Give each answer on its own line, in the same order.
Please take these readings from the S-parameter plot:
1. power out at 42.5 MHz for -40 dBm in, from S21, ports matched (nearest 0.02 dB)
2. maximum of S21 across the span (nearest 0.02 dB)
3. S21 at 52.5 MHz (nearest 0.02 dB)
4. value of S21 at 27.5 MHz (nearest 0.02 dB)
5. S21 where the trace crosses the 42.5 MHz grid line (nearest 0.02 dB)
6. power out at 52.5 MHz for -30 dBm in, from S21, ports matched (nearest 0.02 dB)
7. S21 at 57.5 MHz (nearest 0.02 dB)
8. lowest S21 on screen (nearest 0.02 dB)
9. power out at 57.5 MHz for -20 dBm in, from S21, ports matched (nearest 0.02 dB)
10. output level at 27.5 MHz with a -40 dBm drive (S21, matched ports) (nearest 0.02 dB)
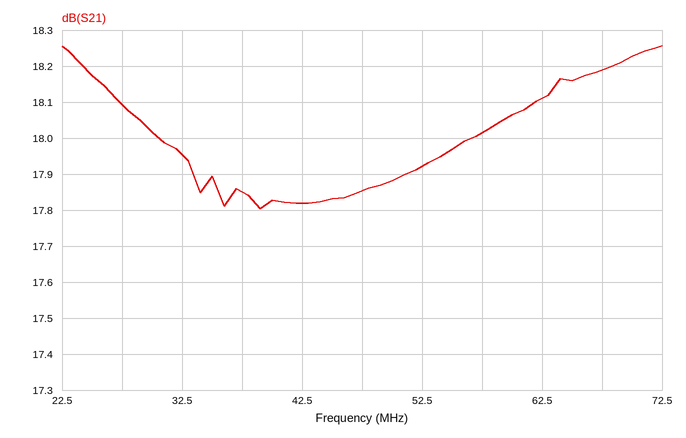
-22.18 dBm
18.26 dB
17.92 dB
18.10 dB
17.82 dB
-12.08 dBm
18.02 dB
17.80 dB
-1.98 dBm
-21.90 dBm
